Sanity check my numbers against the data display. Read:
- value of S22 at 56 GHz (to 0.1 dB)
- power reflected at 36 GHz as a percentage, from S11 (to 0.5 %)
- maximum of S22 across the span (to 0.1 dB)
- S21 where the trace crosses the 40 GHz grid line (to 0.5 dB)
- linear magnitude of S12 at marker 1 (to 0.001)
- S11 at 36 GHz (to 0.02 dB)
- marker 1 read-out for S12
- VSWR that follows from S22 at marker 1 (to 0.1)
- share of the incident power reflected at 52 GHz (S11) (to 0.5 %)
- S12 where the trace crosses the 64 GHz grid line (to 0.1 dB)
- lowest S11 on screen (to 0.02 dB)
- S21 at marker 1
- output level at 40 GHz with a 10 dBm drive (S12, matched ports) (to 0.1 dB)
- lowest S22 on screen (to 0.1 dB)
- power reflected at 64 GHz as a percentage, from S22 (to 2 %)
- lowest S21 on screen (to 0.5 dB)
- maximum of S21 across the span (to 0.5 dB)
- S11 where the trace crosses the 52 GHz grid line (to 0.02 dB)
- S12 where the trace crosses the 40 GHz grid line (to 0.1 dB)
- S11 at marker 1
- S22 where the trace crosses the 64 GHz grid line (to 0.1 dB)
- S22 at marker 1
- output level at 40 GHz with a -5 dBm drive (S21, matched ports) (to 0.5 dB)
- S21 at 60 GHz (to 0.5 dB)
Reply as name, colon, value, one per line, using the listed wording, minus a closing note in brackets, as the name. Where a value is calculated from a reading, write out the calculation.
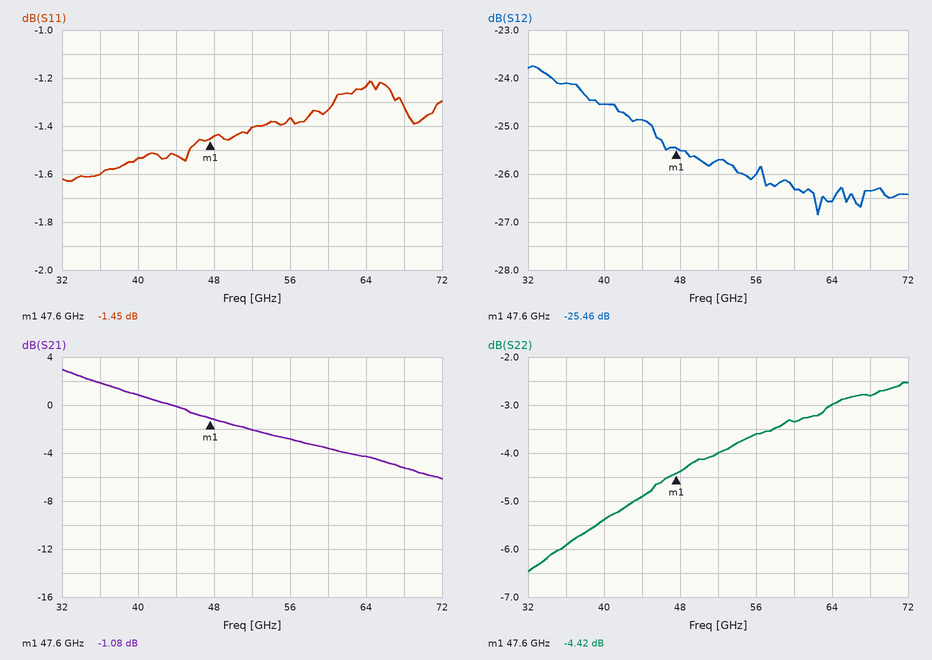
value of S22 at 56 GHz: -3.6 dB
power reflected at 36 GHz as a percentage, from S11: 10^(-1.6/10) ≈ 69.2 %, so 69.0 % to the nearest 0.5 %
maximum of S22 across the span: -2.5 dB
S21 where the trace crosses the 40 GHz grid line: 1.0 dB
linear magnitude of S12 at marker 1: 10^(-25.46/20) ≈ 0.053
S11 at 36 GHz: -1.60 dB
marker 1 read-out for S12: -25.46 dB
VSWR that follows from S22 at marker 1: (1 + 0.6012)/(1 − 0.6012) ≈ 4.0
share of the incident power reflected at 52 GHz (S11): 10^(-1.4/10) ≈ 72.4 %, so 72.5 % to the nearest 0.5 %
S12 where the trace crosses the 64 GHz grid line: -26.6 dB
lowest S11 on screen: -1.62 dB
S21 at marker 1: -1.08 dB
output level at 40 GHz with a 10 dBm drive (S12, matched ports): 10 dBm + (-24.5 dB) = -14.5 dBm
lowest S22 on screen: -6.5 dB
power reflected at 64 GHz as a percentage, from S22: 10^(-3/10) ≈ 50 %
lowest S21 on screen: -6.0 dB
maximum of S21 across the span: 3.0 dB
S11 where the trace crosses the 52 GHz grid line: -1.40 dB
S12 where the trace crosses the 40 GHz grid line: -24.5 dB
S11 at marker 1: -1.45 dB
S22 where the trace crosses the 64 GHz grid line: -3.0 dB
S22 at marker 1: -4.42 dB
output level at 40 GHz with a -5 dBm drive (S21, matched ports): -5 dBm + (1.0 dB) = -4.0 dBm
S21 at 60 GHz: -3.5 dB
